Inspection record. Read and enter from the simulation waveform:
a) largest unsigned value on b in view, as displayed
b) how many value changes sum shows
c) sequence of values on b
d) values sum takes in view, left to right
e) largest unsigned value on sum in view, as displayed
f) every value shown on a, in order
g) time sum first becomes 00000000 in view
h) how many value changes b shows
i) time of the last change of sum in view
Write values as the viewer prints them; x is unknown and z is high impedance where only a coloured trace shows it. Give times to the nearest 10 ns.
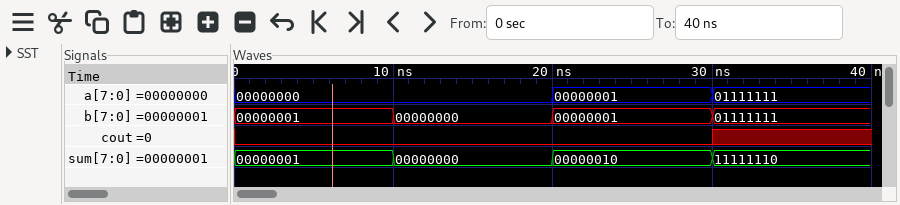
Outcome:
01111111
3
00000001, 00000000, 00000001, 01111111
00000001, 00000000, 00000010, 11111110
11111110
00000000, 00000001, 01111111
10 ns
3
30 ns
